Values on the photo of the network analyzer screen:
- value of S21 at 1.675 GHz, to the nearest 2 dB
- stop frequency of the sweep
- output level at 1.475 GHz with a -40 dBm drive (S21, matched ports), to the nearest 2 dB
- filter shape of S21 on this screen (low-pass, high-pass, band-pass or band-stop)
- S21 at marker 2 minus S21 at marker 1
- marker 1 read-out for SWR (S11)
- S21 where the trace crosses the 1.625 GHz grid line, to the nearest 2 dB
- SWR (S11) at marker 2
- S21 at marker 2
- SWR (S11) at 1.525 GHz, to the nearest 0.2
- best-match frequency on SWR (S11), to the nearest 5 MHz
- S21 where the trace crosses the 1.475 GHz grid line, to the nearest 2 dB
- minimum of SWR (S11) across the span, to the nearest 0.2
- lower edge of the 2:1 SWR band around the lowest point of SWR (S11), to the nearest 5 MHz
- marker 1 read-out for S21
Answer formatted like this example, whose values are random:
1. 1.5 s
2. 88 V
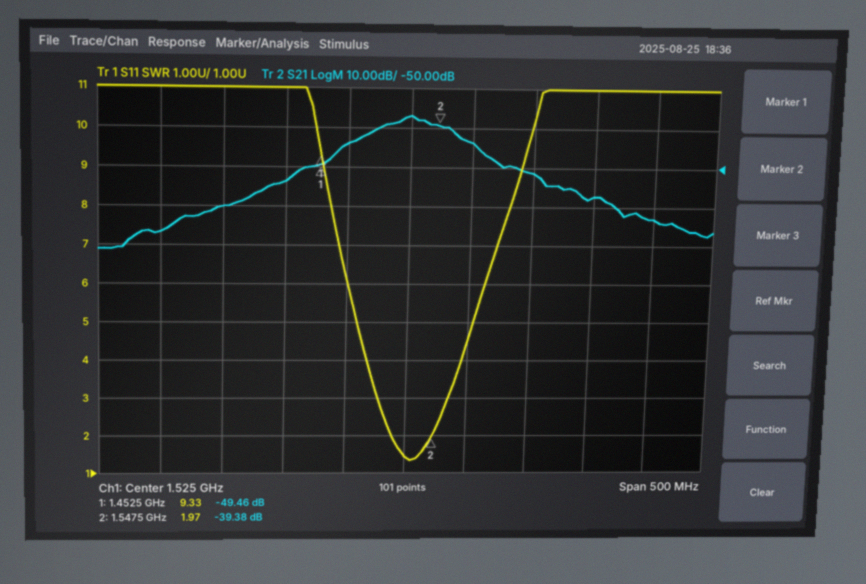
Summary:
1. -58 dB
2. 1.775 GHz
3. -84 dBm
4. band-pass
5. 10.08 dB
6. 9.33
7. -52 dB
8. 1.97
9. -39.38 dB
10. 1.4
11. 1.530 GHz
12. -44 dB
13. 1.4
14. 1.515 GHz
15. -49.46 dB
